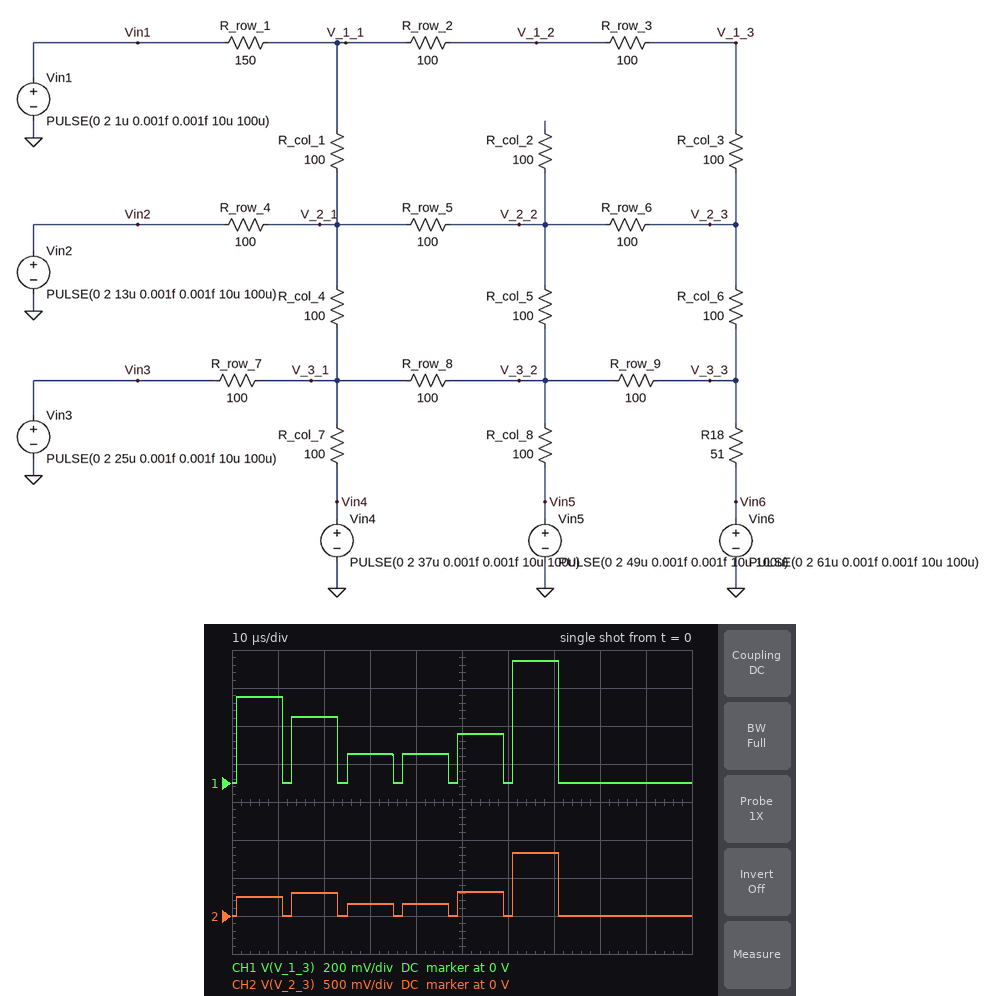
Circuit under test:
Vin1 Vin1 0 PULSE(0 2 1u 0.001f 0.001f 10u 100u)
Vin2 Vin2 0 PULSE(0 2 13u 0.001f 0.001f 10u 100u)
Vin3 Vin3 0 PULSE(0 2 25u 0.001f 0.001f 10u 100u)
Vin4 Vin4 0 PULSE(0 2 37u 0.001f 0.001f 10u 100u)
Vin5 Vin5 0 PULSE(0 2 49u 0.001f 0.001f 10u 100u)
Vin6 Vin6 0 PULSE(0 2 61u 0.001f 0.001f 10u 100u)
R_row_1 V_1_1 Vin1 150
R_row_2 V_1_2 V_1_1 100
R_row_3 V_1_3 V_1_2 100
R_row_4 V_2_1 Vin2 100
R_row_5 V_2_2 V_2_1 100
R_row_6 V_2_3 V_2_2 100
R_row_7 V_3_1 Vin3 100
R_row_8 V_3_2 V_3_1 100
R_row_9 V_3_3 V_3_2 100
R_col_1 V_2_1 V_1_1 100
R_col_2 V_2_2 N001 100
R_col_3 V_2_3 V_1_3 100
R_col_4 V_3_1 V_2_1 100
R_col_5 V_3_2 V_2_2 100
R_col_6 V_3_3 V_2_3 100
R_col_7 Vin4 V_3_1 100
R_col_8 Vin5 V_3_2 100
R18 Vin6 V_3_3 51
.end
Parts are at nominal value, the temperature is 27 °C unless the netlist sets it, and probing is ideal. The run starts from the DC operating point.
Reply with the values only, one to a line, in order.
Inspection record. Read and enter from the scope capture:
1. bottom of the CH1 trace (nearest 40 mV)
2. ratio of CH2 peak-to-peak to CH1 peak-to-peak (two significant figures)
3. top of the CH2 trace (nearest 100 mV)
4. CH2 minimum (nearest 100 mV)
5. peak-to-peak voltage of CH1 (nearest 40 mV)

0 V
1.3
800 mV
0 V
640 mV
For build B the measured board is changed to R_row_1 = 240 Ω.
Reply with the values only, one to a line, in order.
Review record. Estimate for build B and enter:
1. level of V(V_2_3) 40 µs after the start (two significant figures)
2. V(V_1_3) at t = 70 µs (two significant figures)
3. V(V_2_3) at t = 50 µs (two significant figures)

160 mV
670 mV
320 mV
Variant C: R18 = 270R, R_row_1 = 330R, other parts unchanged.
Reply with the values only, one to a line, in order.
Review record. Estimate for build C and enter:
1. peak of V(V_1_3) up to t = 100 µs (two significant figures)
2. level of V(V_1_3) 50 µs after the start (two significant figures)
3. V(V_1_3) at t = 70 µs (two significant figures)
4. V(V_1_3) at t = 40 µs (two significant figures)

500 mV
440 mV
280 mV
240 mV
